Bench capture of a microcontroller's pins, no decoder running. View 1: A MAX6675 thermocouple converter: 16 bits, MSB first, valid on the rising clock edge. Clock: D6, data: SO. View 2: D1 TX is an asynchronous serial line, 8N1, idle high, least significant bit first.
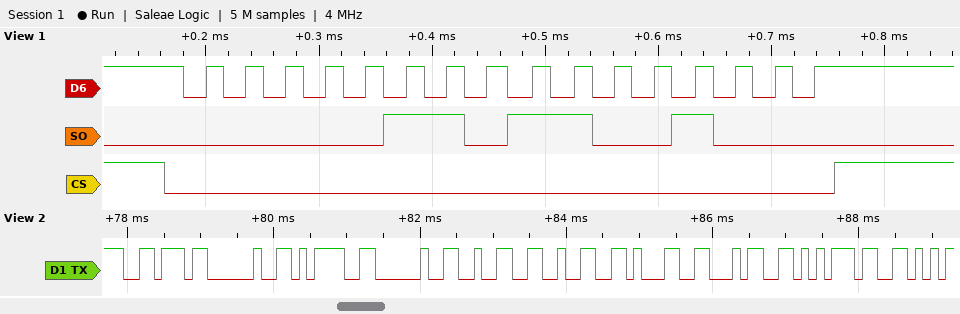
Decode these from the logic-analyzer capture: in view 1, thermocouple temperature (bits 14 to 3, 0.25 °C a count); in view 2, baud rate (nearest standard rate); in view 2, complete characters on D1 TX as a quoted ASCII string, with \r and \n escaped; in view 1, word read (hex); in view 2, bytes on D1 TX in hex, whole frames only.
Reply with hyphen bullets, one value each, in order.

- 54.25 °C
- 9600 baud
- "v = 2214uV"
- 0x06C8
- 76 20 3D 20 32 32 31 34 75 56
